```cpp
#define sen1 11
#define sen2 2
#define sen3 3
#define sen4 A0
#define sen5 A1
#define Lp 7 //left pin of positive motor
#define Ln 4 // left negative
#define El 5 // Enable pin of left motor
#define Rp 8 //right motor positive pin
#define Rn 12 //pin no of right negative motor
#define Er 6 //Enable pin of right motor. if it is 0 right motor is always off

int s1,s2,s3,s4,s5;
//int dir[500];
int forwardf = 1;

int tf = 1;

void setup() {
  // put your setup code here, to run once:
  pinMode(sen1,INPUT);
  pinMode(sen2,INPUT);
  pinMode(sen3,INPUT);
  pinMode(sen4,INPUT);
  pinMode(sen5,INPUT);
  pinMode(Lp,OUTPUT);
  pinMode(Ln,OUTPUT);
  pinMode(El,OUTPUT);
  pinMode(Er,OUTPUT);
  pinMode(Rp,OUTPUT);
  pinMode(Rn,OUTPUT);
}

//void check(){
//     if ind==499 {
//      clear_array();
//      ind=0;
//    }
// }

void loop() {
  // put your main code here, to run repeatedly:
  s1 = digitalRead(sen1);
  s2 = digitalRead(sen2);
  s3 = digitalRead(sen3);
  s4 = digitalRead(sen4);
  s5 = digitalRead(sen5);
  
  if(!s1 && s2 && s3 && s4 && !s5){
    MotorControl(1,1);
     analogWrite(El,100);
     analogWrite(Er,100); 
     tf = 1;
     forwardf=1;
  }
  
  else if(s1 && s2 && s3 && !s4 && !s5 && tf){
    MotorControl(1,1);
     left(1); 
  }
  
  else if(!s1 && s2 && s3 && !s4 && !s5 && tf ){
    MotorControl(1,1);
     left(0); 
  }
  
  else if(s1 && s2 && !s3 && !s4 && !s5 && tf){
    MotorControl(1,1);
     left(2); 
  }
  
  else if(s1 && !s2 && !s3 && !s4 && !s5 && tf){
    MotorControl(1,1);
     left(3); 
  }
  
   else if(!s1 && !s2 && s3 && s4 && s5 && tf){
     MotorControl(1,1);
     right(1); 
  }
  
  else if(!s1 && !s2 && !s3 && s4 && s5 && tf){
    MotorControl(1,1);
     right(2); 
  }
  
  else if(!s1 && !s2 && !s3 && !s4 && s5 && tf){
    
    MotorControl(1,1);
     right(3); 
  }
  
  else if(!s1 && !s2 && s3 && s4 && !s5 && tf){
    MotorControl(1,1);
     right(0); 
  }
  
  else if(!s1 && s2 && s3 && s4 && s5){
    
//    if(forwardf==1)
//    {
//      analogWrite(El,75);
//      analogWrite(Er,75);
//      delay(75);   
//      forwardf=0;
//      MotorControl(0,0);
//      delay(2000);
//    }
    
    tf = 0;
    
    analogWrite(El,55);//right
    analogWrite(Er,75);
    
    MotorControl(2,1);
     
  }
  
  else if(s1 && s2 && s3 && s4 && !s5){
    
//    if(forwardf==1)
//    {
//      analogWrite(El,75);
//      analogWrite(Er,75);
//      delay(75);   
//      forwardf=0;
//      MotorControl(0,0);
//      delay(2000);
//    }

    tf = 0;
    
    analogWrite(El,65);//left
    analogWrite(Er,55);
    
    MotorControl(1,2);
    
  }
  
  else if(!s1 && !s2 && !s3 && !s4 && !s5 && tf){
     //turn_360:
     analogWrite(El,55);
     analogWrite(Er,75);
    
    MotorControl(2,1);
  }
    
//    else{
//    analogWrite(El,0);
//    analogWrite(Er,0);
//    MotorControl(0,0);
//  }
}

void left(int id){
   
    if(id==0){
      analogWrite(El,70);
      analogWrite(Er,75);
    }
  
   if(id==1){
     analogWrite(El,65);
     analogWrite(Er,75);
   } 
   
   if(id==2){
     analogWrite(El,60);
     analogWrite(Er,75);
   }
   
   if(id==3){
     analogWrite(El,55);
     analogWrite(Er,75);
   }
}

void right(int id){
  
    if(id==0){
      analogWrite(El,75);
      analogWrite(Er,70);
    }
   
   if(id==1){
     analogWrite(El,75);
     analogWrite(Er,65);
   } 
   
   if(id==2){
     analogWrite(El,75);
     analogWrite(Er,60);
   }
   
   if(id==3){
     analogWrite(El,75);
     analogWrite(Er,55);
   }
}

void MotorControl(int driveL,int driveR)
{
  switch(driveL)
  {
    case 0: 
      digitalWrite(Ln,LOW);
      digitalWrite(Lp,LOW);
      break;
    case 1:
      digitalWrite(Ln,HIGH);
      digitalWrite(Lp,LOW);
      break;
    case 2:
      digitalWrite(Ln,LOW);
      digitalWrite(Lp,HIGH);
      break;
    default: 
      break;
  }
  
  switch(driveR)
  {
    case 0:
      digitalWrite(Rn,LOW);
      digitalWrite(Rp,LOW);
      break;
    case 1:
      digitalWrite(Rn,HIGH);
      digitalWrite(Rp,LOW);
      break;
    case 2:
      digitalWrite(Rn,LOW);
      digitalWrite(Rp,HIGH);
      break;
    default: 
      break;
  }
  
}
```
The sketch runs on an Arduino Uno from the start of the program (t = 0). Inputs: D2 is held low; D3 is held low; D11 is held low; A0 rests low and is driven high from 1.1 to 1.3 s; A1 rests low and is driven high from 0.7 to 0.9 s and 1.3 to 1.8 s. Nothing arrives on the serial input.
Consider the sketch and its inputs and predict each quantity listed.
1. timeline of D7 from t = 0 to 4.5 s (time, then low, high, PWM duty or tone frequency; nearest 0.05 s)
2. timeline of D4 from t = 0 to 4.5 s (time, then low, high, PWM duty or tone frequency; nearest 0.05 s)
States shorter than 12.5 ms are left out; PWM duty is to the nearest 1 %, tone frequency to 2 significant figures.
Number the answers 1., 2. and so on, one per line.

1. 0 s high; 0.7 s low; 0.9 s high; 1.3 s low; 1.8 s high
2. 0 s low; 0.7 s high; 0.9 s low; 1.3 s high; 1.8 s low
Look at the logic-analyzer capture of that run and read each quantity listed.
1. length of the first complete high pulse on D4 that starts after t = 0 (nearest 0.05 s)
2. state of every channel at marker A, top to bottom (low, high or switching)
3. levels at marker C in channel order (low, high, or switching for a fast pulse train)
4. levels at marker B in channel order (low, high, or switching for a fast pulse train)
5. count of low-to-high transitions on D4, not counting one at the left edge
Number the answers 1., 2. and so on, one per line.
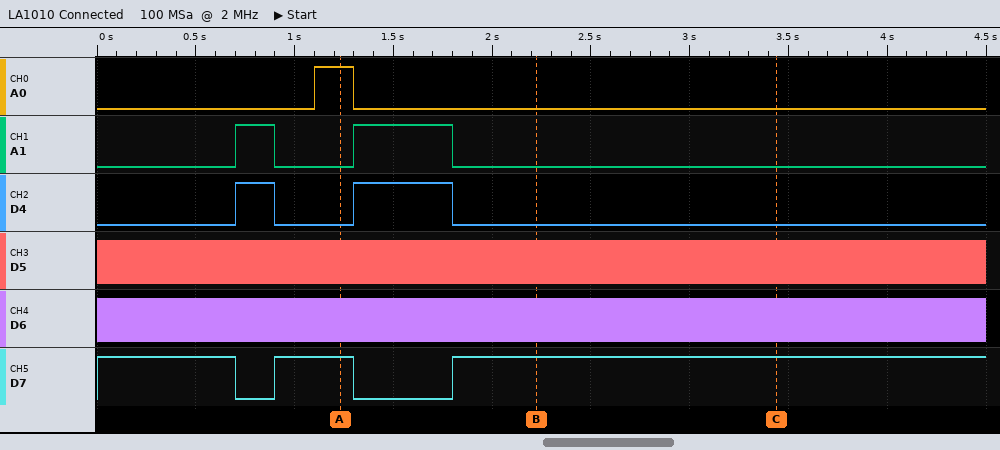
1. 0.20 s
2. A0 high, A1 low, D4 low, D5 switching, D6 switching, D7 high
3. A0 low, A1 low, D4 low, D5 switching, D6 switching, D7 high
4. A0 low, A1 low, D4 low, D5 switching, D6 switching, D7 high
5. 2
